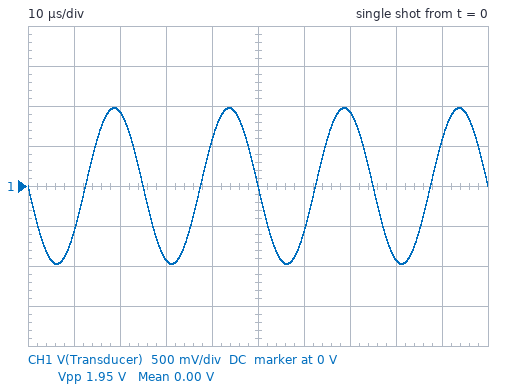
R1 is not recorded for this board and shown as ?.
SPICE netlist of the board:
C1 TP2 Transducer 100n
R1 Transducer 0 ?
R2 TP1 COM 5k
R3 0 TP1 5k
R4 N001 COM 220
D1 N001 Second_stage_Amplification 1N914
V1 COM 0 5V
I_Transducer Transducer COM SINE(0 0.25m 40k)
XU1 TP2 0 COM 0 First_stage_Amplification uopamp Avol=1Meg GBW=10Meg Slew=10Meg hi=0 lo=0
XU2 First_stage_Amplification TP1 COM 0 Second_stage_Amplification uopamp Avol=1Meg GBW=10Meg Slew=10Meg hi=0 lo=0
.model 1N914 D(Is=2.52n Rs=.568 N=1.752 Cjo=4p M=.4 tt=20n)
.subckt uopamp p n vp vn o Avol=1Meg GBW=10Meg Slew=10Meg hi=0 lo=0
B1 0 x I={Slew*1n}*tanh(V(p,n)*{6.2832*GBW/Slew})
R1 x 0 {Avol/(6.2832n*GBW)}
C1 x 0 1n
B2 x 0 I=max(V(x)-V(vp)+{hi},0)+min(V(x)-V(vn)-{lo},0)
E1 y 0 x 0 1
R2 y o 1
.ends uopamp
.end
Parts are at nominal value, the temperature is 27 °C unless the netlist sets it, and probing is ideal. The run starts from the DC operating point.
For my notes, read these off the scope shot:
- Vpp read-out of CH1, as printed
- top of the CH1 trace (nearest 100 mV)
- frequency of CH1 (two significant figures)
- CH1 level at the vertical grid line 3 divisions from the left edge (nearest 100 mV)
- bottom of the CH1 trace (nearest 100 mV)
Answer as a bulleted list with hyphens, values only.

- 1.95 V
- 1.0 V
- 40 kHz
- -900 mV
- -1.0 V
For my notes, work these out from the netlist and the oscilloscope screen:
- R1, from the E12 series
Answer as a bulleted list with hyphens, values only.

- 3.9 kΩ
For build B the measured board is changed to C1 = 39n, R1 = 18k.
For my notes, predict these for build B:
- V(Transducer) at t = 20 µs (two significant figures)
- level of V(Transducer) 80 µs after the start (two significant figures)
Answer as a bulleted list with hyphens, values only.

- 4.3 V
- -4.3 V
